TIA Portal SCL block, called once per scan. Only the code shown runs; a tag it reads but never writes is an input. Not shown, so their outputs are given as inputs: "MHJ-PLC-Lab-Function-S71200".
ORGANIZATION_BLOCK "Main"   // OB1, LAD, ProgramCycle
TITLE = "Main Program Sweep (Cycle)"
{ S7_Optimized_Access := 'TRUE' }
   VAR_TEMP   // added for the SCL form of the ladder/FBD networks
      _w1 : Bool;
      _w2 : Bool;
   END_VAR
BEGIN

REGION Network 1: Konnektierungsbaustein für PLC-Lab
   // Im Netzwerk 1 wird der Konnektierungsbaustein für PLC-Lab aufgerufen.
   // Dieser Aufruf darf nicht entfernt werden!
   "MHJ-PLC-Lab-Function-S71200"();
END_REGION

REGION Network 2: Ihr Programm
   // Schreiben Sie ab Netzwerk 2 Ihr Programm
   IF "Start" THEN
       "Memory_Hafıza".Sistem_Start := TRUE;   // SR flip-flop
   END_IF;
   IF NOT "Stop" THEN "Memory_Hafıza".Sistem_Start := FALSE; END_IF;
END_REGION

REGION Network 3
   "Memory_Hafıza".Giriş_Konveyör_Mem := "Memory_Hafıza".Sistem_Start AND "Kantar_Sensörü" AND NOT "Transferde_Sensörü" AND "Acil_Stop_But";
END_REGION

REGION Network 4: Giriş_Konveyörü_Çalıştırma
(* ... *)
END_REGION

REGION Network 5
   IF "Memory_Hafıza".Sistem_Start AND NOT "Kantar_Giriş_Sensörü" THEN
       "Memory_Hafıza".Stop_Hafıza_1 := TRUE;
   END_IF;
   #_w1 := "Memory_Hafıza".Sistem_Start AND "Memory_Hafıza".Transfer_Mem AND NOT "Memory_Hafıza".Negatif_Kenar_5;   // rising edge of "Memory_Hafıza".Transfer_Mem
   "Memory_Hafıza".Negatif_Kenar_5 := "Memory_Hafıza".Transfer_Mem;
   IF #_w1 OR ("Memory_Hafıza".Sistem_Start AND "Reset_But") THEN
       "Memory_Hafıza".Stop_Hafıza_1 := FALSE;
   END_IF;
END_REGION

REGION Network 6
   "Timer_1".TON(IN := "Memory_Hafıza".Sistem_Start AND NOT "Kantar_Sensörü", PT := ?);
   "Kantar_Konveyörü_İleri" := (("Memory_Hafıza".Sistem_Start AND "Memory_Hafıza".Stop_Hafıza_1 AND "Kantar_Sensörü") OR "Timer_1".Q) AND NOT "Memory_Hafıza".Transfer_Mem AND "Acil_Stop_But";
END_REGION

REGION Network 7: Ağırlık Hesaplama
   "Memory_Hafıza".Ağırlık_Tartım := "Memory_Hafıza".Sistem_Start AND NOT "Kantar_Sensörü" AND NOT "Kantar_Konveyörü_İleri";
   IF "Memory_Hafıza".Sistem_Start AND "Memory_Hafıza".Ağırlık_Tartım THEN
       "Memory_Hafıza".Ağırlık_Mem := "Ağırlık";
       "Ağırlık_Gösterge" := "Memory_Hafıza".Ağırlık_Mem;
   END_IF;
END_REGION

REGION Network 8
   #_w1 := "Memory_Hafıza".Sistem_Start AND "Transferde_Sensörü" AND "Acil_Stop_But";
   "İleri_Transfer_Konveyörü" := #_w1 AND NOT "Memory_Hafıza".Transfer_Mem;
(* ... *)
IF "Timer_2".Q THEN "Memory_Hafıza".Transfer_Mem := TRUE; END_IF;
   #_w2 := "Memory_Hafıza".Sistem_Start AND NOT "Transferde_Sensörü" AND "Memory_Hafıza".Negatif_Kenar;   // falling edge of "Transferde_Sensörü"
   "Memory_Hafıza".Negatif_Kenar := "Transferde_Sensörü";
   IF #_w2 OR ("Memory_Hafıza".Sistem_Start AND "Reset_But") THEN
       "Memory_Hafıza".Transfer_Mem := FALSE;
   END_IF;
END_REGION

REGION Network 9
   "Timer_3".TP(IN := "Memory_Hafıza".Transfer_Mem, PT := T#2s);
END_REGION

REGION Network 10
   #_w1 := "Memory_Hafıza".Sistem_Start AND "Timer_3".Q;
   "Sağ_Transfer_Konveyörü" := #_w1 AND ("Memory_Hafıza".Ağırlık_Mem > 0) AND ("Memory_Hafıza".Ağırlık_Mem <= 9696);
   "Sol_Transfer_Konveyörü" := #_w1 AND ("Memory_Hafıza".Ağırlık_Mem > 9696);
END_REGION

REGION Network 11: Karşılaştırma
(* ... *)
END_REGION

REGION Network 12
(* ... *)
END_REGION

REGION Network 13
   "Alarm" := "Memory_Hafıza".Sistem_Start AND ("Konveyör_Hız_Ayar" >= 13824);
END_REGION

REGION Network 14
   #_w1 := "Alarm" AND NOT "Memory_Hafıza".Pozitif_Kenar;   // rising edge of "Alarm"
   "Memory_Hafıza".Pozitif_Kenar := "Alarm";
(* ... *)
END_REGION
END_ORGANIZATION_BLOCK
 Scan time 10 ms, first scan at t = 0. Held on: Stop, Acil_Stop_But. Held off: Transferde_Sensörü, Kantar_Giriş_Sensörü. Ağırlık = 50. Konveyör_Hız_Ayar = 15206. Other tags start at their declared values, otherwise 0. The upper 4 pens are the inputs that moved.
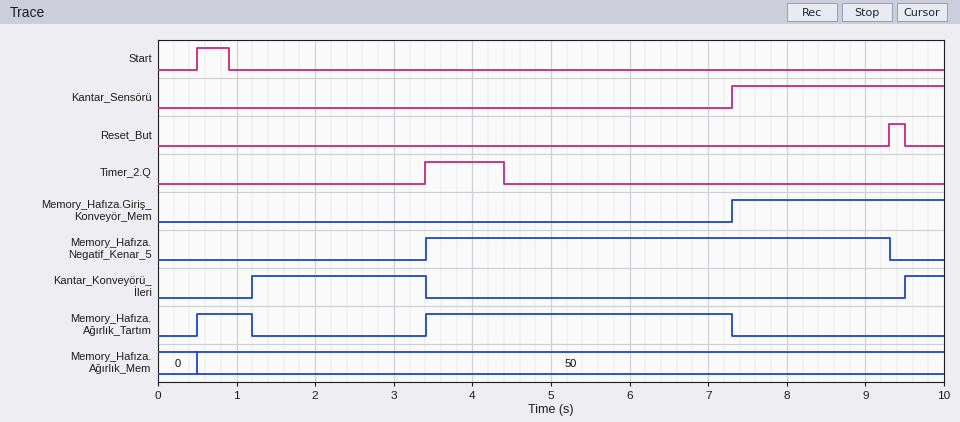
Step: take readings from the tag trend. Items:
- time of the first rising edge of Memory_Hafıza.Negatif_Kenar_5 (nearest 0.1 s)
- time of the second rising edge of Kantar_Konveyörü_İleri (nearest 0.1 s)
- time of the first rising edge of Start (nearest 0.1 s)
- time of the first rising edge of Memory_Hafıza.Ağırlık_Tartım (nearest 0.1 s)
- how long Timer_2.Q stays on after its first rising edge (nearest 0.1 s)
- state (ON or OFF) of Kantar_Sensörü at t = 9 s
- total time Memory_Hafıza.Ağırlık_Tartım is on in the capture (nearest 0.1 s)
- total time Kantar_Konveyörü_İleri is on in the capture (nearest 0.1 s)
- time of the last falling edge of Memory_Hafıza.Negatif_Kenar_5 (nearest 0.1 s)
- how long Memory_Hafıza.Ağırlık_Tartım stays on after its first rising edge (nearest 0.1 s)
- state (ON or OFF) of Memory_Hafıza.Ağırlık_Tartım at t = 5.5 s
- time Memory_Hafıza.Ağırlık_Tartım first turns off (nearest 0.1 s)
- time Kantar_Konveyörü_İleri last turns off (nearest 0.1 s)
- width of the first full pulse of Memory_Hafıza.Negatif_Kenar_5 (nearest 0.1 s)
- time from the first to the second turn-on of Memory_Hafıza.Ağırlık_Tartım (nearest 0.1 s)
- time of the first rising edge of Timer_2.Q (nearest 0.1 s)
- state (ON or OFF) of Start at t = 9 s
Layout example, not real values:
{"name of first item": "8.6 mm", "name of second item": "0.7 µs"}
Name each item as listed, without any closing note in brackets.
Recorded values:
{"time of the first rising edge of Memory_Hafıza.Negatif_Kenar_5": "3.4 s", "time of the second rising edge of Kantar_Konveyörü_İleri": "9.5 s", "time of the first rising edge of Start": "0.5 s", "time of the first rising edge of Memory_Hafıza.Ağırlık_Tartım": "0.5 s", "how long Timer_2.Q stays on after its first rising edge": "1.0 s", "state (ON or OFF) of Kantar_Sensörü at t = 9 s": "ON", "total time Memory_Hafıza.Ağırlık_Tartım is on in the capture": "4.6 s", "total time Kantar_Konveyörü_İleri is on in the capture": "2.7 s", "time of the last falling edge of Memory_Hafıza.Negatif_Kenar_5": "9.3 s", "how long Memory_Hafıza.Ağırlık_Tartım stays on after its first rising edge": "0.7 s", "state (ON or OFF) of Memory_Hafıza.Ağırlık_Tartım at t = 5.5 s": "ON", "time Memory_Hafıza.Ağırlık_Tartım first turns off": "1.2 s", "time Kantar_Konveyörü_İleri last turns off": "3.4 s", "width of the first full pulse of Memory_Hafıza.Negatif_Kenar_5": "5.9 s", "time from the first to the second turn-on of Memory_Hafıza.Ağırlık_Tartım": "2.9 s", "time of the first rising edge of Timer_2.Q": "3.4 s", "state (ON or OFF) of Start at t = 9 s": "OFF"}
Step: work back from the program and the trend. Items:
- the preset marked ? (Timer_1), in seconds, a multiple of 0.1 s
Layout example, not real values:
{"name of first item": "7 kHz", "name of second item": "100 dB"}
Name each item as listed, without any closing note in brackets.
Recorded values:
{"the preset marked ? (Timer_1), in seconds, a multiple of 0.1 s": "0.7 s"}
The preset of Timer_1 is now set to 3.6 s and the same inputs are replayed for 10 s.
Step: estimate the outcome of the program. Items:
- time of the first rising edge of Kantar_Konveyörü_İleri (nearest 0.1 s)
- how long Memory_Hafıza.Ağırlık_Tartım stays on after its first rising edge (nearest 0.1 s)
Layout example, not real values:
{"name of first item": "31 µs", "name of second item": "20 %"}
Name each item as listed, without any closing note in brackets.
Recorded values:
{"time of the first rising edge of Kantar_Konveyörü_İleri": "9.5 s", "how long Memory_Hafıza.Ağırlık_Tartım stays on after its first rising edge": "6.8 s"}
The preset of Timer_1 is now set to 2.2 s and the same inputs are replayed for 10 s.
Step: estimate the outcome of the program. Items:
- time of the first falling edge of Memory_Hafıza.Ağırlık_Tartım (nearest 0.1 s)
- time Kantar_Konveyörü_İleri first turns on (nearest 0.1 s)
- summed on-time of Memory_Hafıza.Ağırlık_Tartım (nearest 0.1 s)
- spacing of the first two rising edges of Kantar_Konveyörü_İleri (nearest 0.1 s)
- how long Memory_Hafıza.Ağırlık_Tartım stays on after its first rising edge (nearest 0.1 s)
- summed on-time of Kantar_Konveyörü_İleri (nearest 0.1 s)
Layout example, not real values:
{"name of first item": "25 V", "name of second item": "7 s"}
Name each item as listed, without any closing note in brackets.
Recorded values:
{"time of the first falling edge of Memory_Hafıza.Ağırlık_Tartım": "2.7 s", "time Kantar_Konveyörü_İleri first turns on": "2.7 s", "summed on-time of Memory_Hafıza.Ağırlık_Tartım": "6.1 s", "spacing of the first two rising edges of Kantar_Konveyörü_İleri": "6.8 s", "how long Memory_Hafıza.Ağırlık_Tartım stays on after its first rising edge": "2.2 s", "summed on-time of Kantar_Konveyörü_İleri": "1.2 s"}
